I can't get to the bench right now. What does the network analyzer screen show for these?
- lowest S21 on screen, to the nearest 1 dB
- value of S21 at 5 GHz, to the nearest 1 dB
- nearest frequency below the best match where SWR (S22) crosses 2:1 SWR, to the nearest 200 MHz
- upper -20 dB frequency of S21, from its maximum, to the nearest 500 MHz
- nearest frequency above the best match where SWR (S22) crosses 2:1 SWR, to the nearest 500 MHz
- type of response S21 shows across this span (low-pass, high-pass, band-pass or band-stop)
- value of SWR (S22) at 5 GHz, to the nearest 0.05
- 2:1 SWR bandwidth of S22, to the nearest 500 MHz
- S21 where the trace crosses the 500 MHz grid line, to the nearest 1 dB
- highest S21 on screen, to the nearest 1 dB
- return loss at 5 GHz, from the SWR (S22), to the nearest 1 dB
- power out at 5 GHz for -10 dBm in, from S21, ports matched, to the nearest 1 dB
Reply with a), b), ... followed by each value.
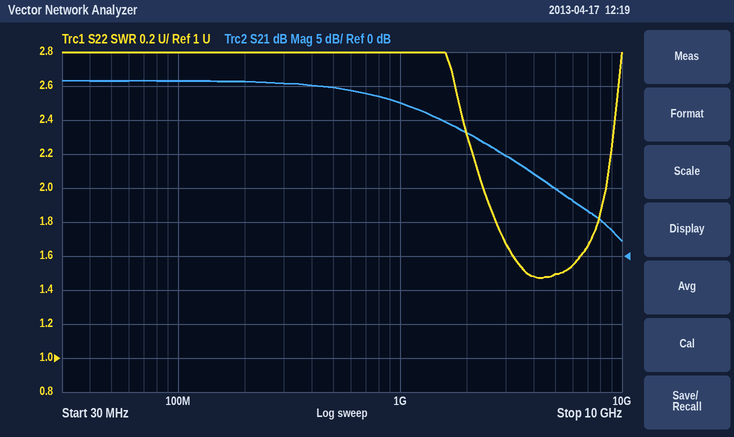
a) 2 dB
b) 10 dB
c) 2.4 GHz
d) 7.5 GHz
e) 8.5 GHz
f) low-pass
g) 1.50
h) 6.0 GHz
i) 25 dB
j) 26 dB
k) 14 dB
l) 0 dBm
